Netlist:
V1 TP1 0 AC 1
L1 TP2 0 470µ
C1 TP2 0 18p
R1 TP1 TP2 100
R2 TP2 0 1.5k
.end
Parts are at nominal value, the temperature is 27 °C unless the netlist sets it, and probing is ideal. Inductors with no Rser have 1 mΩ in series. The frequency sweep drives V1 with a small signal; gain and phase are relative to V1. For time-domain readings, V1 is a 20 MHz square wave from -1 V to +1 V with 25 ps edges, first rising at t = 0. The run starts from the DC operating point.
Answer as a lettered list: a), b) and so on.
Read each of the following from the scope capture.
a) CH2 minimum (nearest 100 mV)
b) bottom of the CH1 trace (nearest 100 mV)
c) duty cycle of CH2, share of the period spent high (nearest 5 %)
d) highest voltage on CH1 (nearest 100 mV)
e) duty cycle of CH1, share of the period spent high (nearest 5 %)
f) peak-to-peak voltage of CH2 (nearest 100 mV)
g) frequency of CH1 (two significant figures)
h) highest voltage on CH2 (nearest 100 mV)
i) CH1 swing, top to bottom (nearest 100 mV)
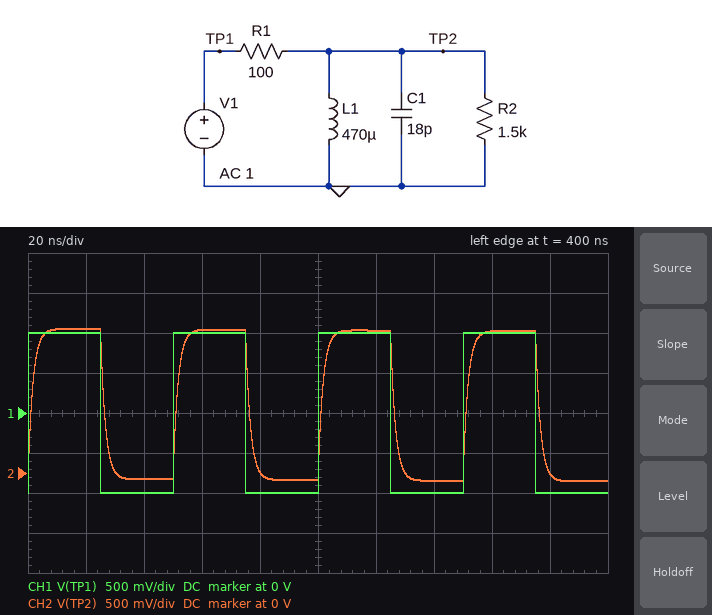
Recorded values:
a) -100 mV
b) -1.0 V
c) 50 %
d) 1.0 V
e) 50 %
f) 1.9 V
g) 20 MHz
h) 1.8 V
i) 2.0 V
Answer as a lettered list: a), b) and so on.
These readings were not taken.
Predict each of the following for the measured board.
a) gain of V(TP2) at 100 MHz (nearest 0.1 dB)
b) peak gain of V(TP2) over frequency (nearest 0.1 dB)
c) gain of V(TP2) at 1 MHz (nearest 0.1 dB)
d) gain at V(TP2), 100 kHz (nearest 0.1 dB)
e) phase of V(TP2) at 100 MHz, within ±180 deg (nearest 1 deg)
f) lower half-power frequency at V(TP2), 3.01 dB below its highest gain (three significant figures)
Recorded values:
a) -3.8 dB
b) -0.6 dB
c) -0.6 dB
d) -1.0 dB
e) -47 deg
f) 31.7 kHz
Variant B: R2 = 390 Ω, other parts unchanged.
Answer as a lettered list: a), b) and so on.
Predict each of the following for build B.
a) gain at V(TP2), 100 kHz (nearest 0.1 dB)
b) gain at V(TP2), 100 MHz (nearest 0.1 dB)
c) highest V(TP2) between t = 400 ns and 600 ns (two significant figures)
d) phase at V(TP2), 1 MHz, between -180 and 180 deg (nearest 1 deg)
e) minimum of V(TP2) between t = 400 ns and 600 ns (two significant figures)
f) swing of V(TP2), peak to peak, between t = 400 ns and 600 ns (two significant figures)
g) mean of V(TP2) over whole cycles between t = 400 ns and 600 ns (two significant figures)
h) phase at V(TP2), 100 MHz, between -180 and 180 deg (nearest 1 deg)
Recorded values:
a) -2.3 dB
b) -4.6 dB
c) 1.5 V
d) 1 deg
e) -77 mV
f) 1.6 V
g) 730 mV
h) -42 deg
